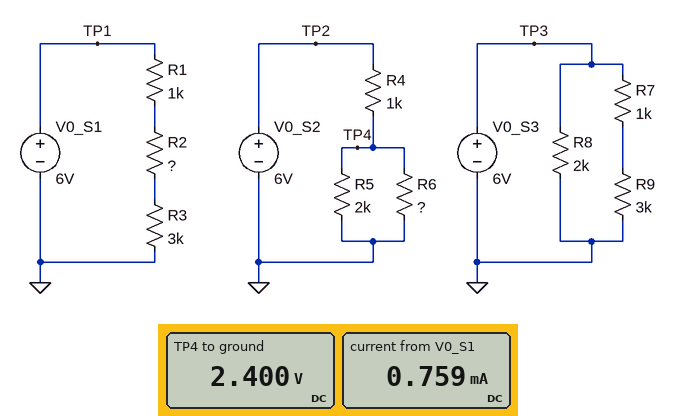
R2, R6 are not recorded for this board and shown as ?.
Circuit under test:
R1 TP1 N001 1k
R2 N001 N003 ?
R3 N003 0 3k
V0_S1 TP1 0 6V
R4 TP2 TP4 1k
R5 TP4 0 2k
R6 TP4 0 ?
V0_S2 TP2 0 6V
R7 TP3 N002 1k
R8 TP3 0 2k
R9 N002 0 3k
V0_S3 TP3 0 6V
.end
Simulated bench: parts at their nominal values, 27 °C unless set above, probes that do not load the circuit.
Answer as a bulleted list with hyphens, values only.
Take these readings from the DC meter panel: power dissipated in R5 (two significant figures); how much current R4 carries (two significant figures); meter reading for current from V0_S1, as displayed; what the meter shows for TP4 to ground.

- 2.9 mW
- 3.6 mA
- 0.759 mA
- 2.400 V
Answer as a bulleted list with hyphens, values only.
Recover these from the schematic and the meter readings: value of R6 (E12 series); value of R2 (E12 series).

- 1 kΩ
- 3.9 kΩ
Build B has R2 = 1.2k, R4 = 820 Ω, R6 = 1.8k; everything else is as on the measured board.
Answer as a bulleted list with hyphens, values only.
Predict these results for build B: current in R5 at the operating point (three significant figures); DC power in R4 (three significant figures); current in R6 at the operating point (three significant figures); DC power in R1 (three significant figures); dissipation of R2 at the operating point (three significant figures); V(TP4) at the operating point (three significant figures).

- 1.61 mA
- 9.45 mW
- 1.79 mA
- 1.33 mW
- 1.60 mW
- 3.22 V
